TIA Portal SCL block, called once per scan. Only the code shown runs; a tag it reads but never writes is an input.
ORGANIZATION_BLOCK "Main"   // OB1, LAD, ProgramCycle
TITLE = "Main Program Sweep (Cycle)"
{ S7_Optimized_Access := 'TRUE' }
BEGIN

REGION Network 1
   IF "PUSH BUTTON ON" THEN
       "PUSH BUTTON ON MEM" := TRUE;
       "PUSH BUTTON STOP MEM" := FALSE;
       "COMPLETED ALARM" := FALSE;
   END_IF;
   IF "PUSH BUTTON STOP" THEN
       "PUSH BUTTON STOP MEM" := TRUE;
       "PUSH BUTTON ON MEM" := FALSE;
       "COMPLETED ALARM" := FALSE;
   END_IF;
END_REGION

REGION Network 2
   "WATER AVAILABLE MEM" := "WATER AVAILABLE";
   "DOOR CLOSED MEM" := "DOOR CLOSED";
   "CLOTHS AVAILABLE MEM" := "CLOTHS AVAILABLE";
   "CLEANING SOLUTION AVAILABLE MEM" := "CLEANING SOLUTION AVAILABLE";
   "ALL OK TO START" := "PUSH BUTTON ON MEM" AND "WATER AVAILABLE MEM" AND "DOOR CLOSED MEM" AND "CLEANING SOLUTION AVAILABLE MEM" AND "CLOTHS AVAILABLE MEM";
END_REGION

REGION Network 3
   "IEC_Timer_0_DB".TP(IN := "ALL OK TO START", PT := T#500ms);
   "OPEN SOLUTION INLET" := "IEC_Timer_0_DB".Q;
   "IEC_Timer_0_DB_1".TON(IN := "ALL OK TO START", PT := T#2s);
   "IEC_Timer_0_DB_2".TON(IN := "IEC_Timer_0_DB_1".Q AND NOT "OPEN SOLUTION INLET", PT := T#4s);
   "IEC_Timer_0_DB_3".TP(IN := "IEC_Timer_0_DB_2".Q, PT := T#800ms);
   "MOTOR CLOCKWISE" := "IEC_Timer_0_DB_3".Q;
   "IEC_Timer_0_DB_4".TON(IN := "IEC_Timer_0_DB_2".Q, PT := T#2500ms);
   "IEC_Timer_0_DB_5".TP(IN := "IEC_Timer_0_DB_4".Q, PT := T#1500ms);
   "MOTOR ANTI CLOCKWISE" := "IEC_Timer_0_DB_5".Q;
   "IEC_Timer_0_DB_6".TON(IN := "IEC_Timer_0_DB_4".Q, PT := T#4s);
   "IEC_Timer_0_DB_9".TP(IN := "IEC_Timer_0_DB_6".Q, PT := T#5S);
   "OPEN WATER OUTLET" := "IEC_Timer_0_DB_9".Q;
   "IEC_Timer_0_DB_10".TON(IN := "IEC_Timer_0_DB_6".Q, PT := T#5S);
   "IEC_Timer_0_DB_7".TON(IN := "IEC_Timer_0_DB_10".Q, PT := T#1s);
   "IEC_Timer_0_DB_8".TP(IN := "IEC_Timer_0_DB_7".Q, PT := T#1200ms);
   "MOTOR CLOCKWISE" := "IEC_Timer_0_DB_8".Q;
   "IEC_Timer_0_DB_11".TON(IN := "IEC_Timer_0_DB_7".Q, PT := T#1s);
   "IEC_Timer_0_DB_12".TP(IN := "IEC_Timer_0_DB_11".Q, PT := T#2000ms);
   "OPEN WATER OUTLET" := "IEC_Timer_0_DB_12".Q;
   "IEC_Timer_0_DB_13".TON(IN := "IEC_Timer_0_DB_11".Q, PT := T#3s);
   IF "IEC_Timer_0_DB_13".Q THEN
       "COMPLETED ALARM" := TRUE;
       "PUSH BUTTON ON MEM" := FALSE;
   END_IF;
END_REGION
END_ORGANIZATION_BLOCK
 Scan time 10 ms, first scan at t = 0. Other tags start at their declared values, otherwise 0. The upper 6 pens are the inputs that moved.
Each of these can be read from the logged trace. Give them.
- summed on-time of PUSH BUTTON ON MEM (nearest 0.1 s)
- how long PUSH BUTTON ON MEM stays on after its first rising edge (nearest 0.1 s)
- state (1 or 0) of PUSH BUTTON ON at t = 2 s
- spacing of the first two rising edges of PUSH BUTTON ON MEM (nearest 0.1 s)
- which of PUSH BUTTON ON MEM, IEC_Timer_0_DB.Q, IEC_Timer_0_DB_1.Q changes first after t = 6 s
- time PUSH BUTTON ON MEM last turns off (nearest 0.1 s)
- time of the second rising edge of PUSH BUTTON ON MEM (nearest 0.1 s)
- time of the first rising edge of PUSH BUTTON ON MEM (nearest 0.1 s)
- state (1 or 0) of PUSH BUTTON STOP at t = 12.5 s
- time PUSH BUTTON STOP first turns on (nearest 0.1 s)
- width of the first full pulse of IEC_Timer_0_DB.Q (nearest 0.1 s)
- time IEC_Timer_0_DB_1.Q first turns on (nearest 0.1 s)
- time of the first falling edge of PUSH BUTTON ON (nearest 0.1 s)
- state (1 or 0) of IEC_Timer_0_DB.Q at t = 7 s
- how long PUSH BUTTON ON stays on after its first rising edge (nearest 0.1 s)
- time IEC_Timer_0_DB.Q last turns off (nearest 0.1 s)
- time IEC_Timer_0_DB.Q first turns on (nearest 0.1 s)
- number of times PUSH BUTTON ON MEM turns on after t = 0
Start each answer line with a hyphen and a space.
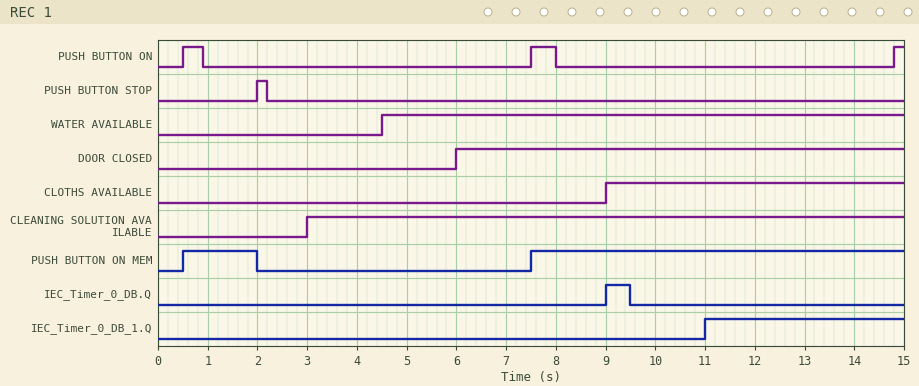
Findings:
- 9.0 s
- 1.5 s
- 0
- 7.0 s
- PUSH BUTTON ON MEM
- 2.0 s
- 7.5 s
- 0.5 s
- 0
- 2.0 s
- 0.5 s
- 11.0 s
- 0.9 s
- 0
- 0.4 s
- 9.5 s
- 9.0 s
- 2
